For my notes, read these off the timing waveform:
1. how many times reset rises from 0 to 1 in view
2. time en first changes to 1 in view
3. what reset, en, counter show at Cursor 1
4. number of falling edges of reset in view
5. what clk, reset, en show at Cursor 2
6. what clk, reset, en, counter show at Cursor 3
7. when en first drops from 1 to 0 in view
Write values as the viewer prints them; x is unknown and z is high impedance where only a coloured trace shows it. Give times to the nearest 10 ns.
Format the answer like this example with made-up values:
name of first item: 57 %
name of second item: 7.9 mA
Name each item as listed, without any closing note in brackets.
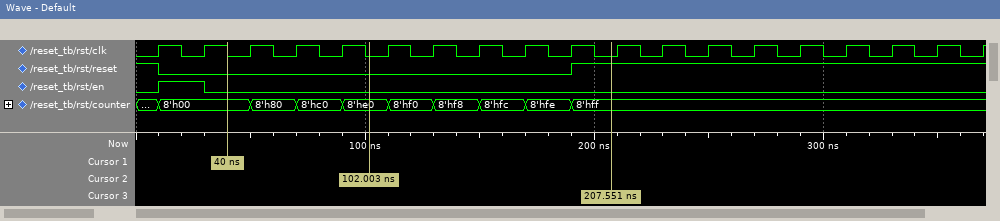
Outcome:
how many times reset rises from 0 to 1 in view: 1
time en first changes to 1 in view: 10 ns
what reset, en, counter show at Cursor 1: reset=0, en=0, counter=8'h00
number of falling edges of reset in view: 1
what clk, reset, en show at Cursor 2: clk=0, reset=0, en=0
what clk, reset, en, counter show at Cursor 3: clk=0, reset=1, en=0, counter=8'hff
when en first drops from 1 to 0 in view: 30 ns
